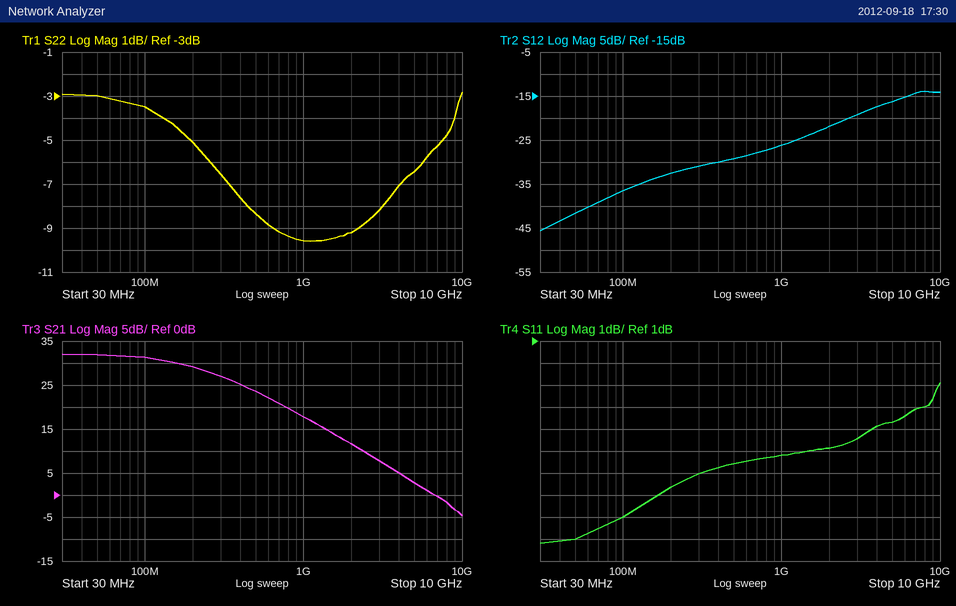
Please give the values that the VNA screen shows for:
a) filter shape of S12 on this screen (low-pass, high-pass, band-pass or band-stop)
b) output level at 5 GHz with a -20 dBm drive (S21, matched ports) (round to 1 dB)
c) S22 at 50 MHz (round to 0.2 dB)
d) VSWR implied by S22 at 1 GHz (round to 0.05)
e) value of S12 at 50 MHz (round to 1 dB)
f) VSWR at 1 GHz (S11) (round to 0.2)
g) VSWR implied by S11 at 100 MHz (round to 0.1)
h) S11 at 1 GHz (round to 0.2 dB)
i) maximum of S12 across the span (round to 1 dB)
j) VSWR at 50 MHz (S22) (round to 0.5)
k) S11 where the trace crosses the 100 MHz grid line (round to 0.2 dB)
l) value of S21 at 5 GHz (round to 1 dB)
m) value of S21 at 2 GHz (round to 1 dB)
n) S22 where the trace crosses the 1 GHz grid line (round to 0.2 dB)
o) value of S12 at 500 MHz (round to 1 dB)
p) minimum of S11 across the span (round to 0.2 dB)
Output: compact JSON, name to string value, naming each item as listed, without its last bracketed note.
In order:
{"filter shape of S12 on this screen": "high-pass", "output level at 5 GHz with a -20 dBm drive (S21, matched ports)": "-17 dBm", "S22 at 50 MHz": "-3.0 dB", "VSWR implied by S22 at 1 GHz": "2.00", "value of S12 at 50 MHz": "-42 dB", "VSWR at 1 GHz (S11)": "4.2", "VSWR implied by S11 at 100 MHz": "2.6", "S11 at 1 GHz": "-4.2 dB", "maximum of S12 across the span": "-14 dB", "VSWR at 50 MHz (S22)": "6.0", "S11 where the trace crosses the 100 MHz grid line": "-7.0 dB", "value of S21 at 5 GHz": "3 dB", "value of S21 at 2 GHz": "12 dB", "S22 where the trace crosses the 1 GHz grid line": "-9.6 dB", "value of S12 at 500 MHz": "-29 dB", "minimum of S11 across the span": "-8.2 dB"}
